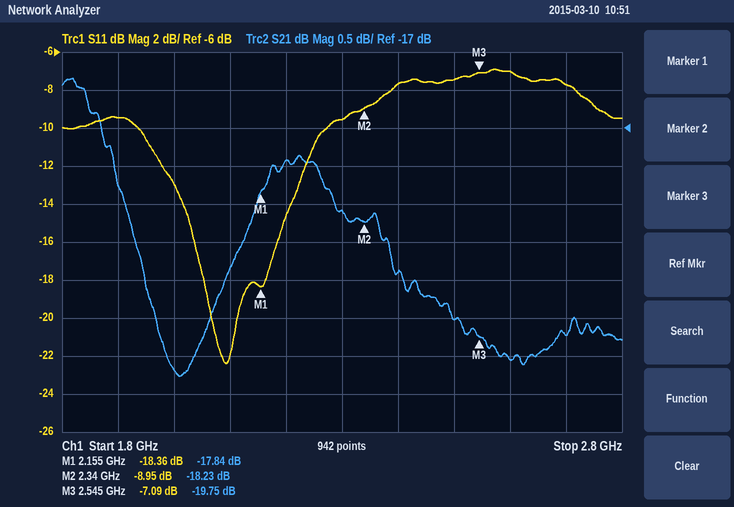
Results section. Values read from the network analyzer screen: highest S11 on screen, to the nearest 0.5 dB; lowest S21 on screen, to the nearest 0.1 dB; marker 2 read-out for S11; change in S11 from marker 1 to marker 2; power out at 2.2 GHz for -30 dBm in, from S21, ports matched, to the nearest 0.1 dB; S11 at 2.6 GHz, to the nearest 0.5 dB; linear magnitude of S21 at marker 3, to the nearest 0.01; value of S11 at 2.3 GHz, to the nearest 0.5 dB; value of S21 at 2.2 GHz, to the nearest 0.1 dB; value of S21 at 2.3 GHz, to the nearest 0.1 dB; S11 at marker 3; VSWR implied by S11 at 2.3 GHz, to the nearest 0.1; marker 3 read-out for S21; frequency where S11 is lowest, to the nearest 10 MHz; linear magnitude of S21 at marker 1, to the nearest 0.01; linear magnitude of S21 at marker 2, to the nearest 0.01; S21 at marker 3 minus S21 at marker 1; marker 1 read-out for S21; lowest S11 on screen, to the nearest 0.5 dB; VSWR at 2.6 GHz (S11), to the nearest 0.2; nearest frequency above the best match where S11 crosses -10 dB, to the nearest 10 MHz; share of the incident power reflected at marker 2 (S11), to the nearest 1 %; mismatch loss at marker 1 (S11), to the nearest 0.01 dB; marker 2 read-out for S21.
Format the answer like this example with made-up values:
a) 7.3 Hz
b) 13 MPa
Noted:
a) -7.0 dB
b) -20.3 dB
c) -8.95 dB
d) 9.41 dB
e) -47.4 dBm
f) -7.0 dB
g) 0.10
h) -9.5 dB
i) -17.4 dB
j) -18.1 dB
k) -7.09 dB
l) 2.0
m) -19.75 dB
n) 2.09 GHz
o) 0.13
p) 0.12
q) -1.91 dB
r) -17.84 dB
s) -22.5 dB
t) 2.6
u) 2.27 GHz
v) 13 %
w) 0.06 dB
x) -18.23 dB
